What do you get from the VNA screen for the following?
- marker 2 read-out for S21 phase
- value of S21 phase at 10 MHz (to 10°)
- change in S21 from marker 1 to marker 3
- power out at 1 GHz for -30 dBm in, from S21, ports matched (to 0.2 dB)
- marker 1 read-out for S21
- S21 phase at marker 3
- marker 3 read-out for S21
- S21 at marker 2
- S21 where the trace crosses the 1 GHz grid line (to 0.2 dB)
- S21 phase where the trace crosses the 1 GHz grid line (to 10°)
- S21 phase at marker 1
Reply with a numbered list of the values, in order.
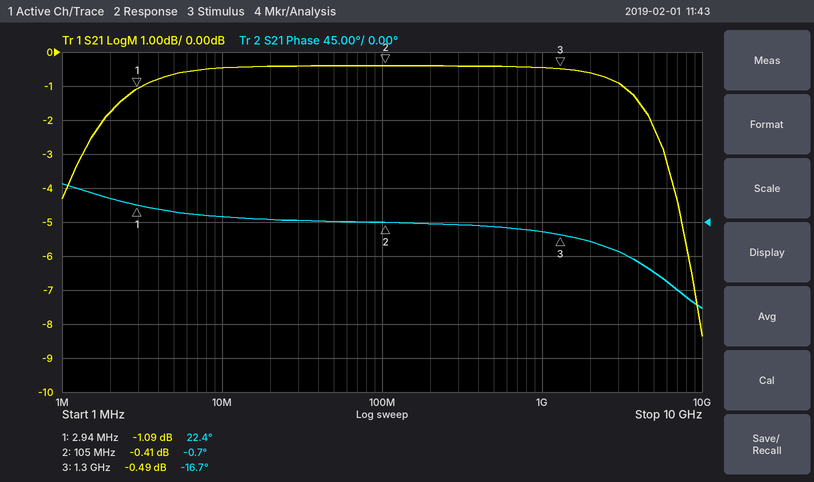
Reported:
1. -0.7°
2. 10°
3. 0.60 dB
4. -30.4 dBm
5. -1.09 dB
6. -16.7°
7. -0.49 dB
8. -0.41 dB
9. -0.4 dB
10. -10°
11. 22.4°
